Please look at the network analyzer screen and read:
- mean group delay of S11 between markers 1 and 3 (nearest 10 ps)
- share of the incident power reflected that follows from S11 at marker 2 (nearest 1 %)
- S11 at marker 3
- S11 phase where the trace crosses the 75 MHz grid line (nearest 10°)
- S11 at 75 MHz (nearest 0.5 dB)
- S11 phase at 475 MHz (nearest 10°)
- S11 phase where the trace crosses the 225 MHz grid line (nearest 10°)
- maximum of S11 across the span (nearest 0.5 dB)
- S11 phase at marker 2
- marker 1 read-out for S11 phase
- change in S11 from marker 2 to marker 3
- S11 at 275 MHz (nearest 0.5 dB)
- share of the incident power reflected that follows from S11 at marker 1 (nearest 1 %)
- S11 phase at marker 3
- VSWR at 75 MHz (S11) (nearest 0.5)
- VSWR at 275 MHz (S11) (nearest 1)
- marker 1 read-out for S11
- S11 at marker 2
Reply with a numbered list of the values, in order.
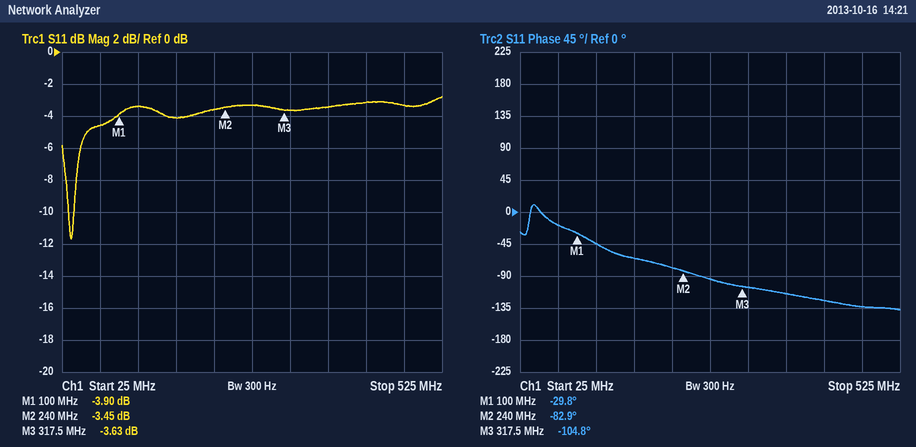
1. 960 ps
2. 45 %
3. -3.63 dB
4. -20°
5. -4.5 dB
6. -130°
7. -80°
8. -3.0 dB
9. -82.9°
10. -29.8°
11. -0.18 dB
12. -3.5 dB
13. 41 %
14. -104.8°
15. 4.0
16. 5
17. -3.90 dB
18. -3.45 dB
